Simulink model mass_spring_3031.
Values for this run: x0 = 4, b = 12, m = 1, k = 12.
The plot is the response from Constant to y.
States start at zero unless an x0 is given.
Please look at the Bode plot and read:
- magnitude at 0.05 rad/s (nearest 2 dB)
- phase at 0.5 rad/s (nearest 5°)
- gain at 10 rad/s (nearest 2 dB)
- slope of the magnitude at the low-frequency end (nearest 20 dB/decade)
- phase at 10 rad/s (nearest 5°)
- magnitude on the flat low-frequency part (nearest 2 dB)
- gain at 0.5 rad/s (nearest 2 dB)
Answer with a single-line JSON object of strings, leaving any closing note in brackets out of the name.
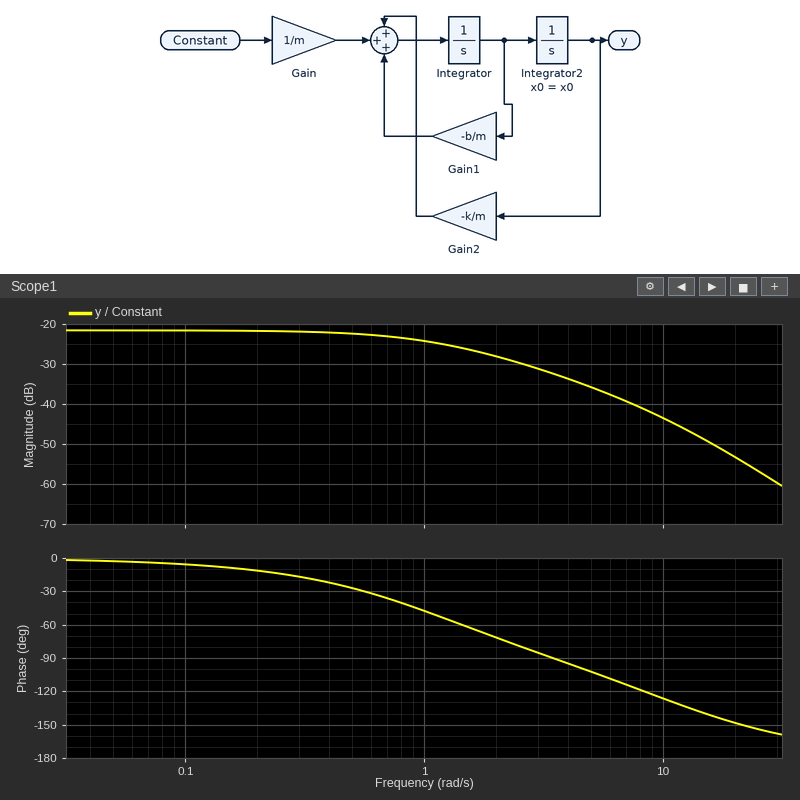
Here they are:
{"magnitude at 0.05 rad/s": "-22 dB", "phase at 0.5 rad/s": "-25°", "gain at 10 rad/s": "-44 dB", "slope of the magnitude at the low-frequency end": "0 dB/decade", "phase at 10 rad/s": "-125°", "magnitude on the flat low-frequency part": "-22 dB", "gain at 0.5 rad/s": "-22 dB"}
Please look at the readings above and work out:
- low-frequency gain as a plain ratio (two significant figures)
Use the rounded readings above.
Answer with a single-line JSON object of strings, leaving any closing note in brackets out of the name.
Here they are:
{"low-frequency gain as a plain ratio": "0.079"}
